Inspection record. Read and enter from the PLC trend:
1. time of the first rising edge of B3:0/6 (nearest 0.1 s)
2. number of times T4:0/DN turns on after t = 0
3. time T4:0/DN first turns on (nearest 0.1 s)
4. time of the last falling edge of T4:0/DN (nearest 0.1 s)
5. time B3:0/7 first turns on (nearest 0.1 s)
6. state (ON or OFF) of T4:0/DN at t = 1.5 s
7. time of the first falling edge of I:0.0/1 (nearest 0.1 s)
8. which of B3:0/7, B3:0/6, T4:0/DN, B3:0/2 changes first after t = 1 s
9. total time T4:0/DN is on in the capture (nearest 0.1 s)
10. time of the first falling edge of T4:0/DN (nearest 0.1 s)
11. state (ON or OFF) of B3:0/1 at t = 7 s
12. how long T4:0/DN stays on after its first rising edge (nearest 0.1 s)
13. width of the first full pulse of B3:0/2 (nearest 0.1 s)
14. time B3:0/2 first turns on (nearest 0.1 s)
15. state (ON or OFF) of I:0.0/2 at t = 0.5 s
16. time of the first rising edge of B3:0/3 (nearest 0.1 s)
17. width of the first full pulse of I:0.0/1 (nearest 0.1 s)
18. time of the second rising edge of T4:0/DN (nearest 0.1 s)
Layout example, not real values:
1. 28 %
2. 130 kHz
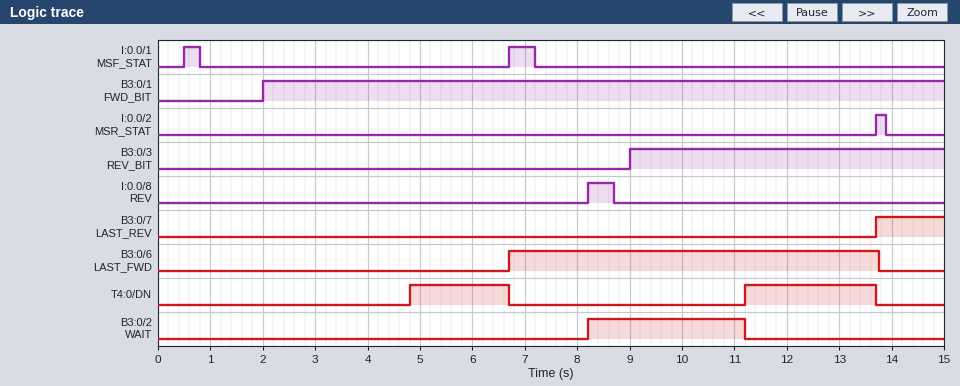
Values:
1. 6.7 s
2. 2
3. 4.8 s
4. 13.7 s
5. 13.7 s
6. OFF
7. 0.8 s
8. T4:0/DN
9. 4.4 s
10. 6.7 s
11. ON
12. 1.9 s
13. 3.0 s
14. 8.2 s
15. OFF
16. 9.0 s
17. 0.3 s
18. 11.2 s
